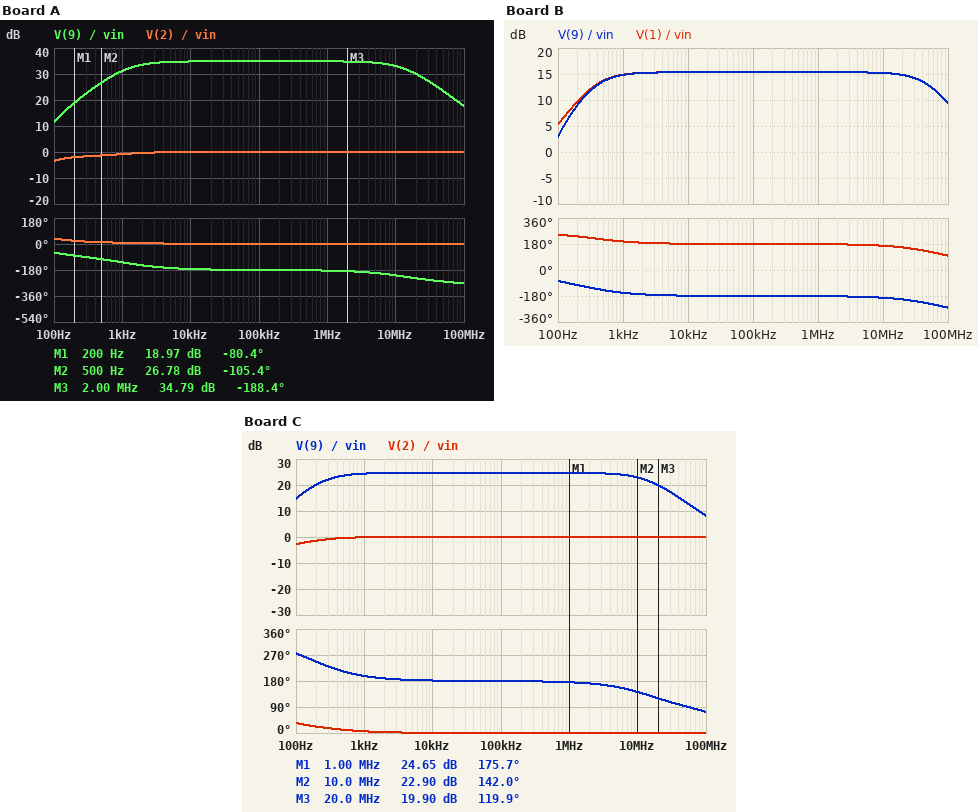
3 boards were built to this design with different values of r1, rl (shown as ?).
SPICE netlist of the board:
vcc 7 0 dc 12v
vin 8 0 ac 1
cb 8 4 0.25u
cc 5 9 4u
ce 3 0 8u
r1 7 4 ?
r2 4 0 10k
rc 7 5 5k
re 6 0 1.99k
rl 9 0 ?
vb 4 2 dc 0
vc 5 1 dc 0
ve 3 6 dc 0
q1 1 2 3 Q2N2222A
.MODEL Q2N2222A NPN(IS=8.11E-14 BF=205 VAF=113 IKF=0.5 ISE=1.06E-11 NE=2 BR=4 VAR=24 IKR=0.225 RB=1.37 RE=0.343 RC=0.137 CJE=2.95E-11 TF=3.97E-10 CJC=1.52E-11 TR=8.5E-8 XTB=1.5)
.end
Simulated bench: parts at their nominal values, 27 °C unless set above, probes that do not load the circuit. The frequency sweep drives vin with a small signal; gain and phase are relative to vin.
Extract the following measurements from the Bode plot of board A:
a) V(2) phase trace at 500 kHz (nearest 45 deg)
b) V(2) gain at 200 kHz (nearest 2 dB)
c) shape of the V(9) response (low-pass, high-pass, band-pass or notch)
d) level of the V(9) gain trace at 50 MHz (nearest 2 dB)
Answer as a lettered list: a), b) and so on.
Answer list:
a) 0 deg
b) 0 dB
c) band-pass
d) 24 dB
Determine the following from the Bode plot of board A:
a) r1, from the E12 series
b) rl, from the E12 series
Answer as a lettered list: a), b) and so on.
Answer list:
a) 27 kΩ
b) 1.5 kΩ
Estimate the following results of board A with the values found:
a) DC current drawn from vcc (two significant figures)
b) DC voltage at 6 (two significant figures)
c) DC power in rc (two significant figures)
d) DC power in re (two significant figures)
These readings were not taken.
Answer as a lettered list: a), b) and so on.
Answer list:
a) 1.6 mA
b) 2.6 V
c) 8.3 mW
d) 3.3 mW
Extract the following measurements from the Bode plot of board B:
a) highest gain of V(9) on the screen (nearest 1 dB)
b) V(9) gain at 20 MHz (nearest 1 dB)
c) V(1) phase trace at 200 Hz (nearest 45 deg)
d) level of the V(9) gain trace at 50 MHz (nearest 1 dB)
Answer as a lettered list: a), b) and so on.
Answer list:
a) 15 dB
b) 15 dB
c) 225 deg
d) 13 dB
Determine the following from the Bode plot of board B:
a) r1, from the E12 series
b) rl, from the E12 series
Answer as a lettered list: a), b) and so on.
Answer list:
a) 82 kΩ
b) 470 Ω
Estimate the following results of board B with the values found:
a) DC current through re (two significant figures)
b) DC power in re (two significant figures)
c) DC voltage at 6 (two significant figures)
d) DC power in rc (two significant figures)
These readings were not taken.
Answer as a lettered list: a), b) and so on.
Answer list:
a) 360 µA
b) 250 µW
c) 710 mV
d) 630 µW
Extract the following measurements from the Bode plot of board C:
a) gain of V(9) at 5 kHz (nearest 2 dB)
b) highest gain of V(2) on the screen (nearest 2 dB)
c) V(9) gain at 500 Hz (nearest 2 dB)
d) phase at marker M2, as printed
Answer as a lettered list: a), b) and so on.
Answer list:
a) 24 dB
b) 0 dB
c) 24 dB
d) 142.0 deg
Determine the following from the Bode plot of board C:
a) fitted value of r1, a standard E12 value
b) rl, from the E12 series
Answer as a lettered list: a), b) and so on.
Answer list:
a) 100 kΩ
b) 2.7 kΩ
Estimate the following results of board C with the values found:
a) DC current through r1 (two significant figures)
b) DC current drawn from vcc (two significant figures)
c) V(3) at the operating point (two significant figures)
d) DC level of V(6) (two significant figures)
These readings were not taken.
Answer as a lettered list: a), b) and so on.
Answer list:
a) 110 µA
b) 360 µA
c) 510 mV
d) 510 mV
